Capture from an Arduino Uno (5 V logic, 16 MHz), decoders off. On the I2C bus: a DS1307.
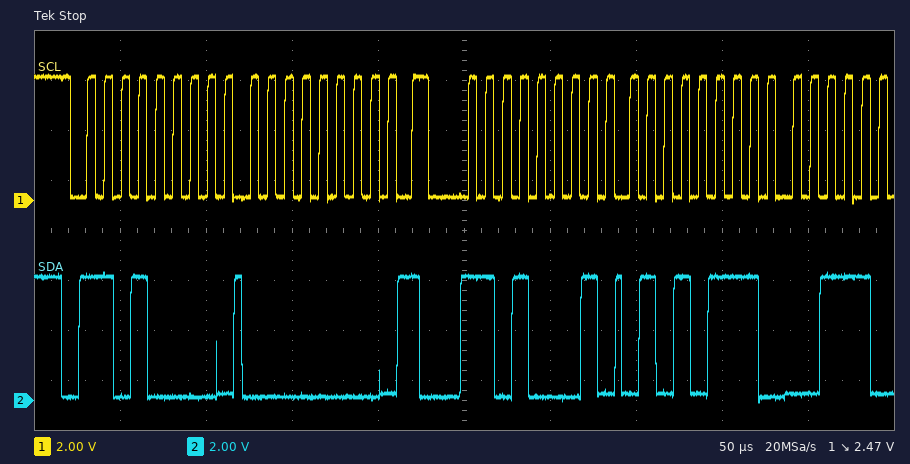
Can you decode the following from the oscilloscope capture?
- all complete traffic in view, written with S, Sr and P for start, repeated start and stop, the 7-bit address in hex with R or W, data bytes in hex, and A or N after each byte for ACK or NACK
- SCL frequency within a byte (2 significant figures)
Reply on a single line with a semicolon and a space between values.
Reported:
S 68W A 00 A Sr 68R A 57 A; 100 kHz
